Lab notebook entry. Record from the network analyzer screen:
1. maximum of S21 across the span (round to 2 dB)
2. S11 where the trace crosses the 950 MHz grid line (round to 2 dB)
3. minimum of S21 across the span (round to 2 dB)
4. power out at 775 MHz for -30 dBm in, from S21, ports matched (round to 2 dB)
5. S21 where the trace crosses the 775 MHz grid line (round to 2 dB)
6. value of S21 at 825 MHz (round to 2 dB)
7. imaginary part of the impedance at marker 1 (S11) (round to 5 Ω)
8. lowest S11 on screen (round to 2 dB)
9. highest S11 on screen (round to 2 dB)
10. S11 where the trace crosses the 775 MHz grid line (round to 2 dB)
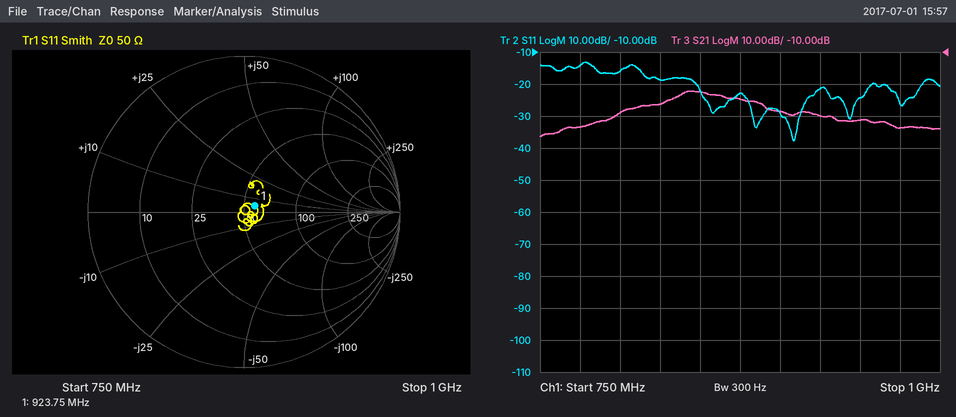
-22 dB
-24 dB
-36 dB
-64 dBm
-34 dB
-26 dB
+5 Ω
-38 dB
-14 dB
-14 dB
